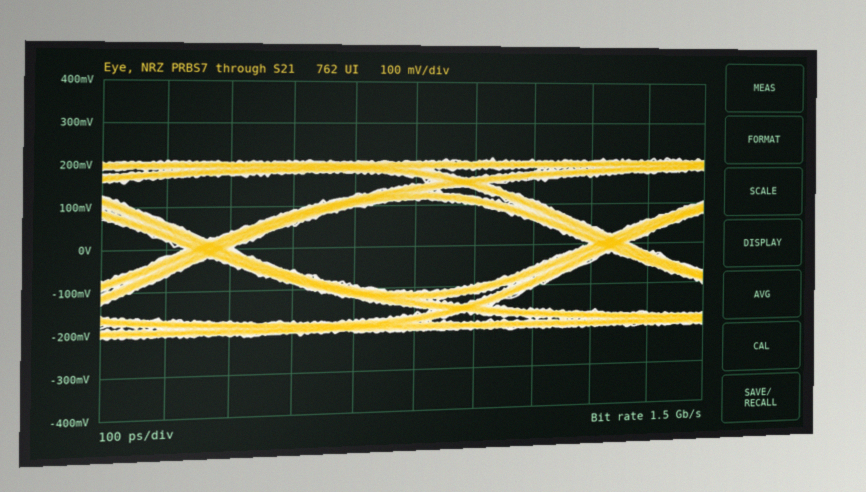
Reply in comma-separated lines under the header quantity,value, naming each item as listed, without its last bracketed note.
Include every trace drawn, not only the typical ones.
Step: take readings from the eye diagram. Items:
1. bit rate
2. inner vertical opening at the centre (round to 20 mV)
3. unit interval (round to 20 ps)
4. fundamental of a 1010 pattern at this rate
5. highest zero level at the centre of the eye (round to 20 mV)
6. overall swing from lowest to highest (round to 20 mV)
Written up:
quantity,value
bit rate,1.5 Gb/s
inner vertical opening at the centre,220 mV
unit interval,660 ps
fundamental of a 1010 pattern at this rate,750 MHz
highest zero level at the centre of the eye,-120 mV
overall swing from lowest to highest,420 mV
